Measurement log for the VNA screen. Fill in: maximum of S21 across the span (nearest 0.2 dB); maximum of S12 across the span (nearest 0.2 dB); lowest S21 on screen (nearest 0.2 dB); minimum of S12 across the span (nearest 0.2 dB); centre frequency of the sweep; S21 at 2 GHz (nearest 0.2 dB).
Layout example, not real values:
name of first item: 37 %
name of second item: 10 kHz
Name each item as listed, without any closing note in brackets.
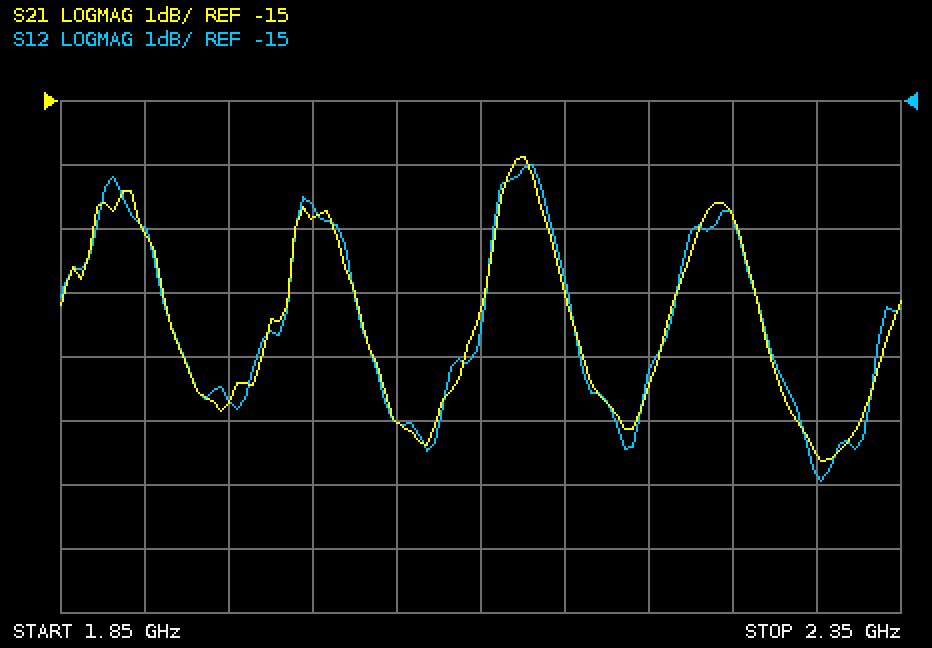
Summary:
maximum of S21 across the span: -15.8 dB
maximum of S12 across the span: -16.0 dB
lowest S21 on screen: -20.6 dB
minimum of S12 across the span: -21.0 dB
centre frequency of the sweep: 2.1 GHz
S21 at 2 GHz: -16.8 dB
